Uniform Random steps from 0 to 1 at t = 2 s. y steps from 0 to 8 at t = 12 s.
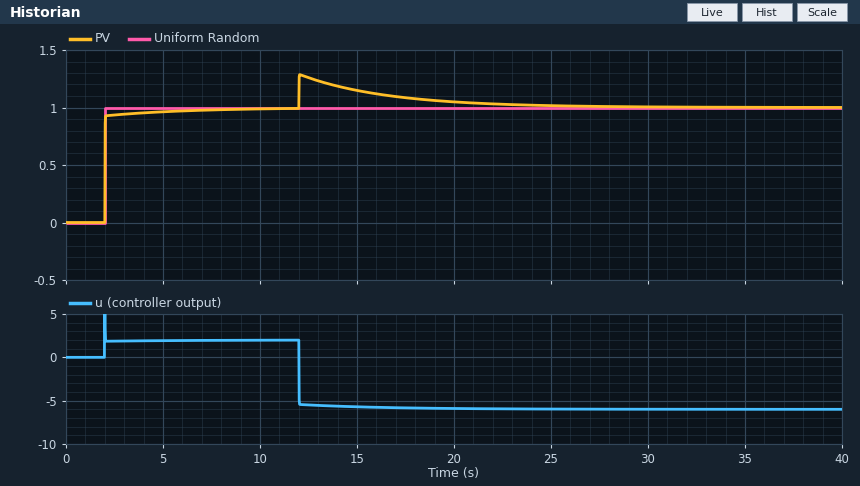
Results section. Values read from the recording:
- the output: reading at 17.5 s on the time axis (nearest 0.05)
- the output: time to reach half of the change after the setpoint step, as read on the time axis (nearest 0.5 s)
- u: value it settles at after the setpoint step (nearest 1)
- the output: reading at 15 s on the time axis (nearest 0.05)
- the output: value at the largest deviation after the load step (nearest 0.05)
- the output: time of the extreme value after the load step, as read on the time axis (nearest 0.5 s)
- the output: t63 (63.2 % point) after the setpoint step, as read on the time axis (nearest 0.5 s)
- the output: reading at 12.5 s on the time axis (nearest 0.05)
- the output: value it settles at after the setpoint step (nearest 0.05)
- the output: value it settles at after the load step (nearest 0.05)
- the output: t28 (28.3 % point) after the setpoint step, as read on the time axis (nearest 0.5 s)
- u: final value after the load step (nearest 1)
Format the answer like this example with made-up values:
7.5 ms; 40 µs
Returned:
1.10; 2.0 s; 2; 1.15; 1.30; 12.0 s; 2.0 s; 1.25; 1.00; 1.00; 2.0 s; -6
